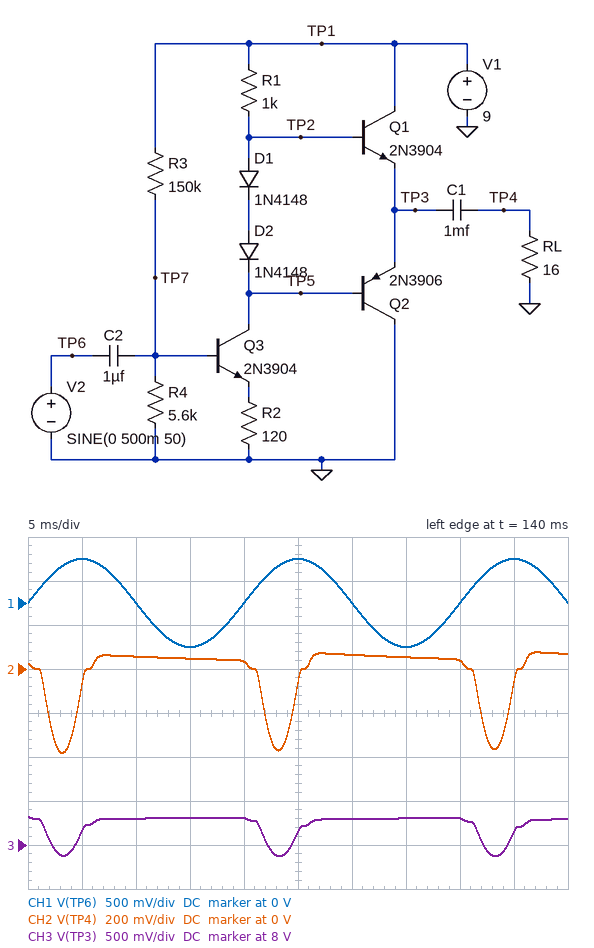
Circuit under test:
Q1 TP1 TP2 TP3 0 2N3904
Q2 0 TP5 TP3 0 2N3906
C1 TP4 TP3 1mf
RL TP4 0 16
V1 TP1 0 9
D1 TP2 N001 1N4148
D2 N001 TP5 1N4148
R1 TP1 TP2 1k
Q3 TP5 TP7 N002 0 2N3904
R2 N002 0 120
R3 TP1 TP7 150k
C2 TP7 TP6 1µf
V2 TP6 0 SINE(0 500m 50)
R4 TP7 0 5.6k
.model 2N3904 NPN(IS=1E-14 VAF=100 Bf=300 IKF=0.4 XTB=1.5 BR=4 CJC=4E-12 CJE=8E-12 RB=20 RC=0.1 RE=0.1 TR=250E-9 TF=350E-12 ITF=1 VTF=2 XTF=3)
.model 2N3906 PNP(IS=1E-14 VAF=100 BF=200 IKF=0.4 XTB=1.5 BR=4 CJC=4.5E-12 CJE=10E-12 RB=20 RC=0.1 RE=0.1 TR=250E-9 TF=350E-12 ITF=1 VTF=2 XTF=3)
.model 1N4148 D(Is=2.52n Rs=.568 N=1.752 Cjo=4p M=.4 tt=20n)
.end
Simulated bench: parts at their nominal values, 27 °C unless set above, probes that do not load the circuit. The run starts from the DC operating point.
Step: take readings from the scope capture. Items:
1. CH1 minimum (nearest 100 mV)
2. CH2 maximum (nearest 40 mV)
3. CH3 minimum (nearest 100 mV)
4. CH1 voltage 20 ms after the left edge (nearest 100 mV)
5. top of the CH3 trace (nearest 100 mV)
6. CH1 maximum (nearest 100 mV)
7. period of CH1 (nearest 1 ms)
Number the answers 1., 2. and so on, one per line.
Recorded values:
1. -500 mV
2. 80 mV
3. 7.9 V
4. 0 V
5. 8.3 V
6. 500 mV
7. 20 ms
